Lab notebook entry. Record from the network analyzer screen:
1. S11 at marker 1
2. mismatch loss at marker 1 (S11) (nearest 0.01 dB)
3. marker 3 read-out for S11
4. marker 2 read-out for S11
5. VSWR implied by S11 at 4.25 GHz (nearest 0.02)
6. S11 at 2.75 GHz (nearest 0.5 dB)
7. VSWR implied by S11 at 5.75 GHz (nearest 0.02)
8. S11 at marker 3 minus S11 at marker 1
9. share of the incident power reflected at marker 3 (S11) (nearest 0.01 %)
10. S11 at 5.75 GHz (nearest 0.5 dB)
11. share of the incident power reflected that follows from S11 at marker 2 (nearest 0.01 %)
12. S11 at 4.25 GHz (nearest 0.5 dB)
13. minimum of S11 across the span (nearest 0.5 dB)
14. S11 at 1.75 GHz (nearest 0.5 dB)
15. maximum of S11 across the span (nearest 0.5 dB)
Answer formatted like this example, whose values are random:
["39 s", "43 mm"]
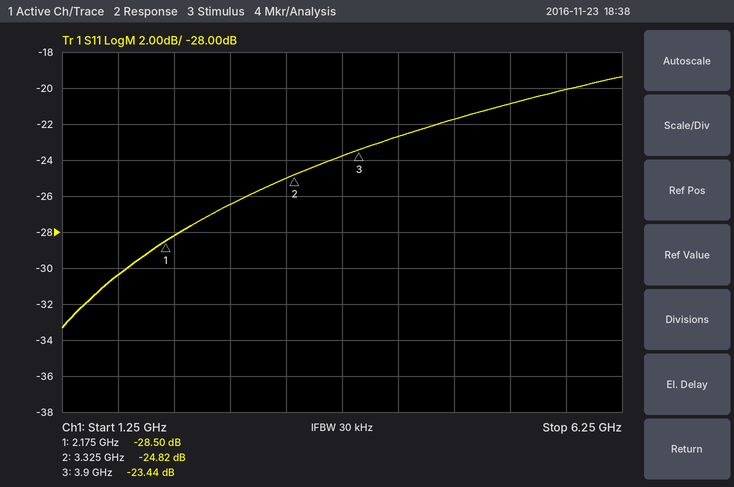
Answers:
["-28.50 dB", "0.01 dB", "-23.44 dB", "-24.82 dB", "1.16", "-26.5 dB", "1.22", "5.06 dB", "0.45 %", "-20.0 dB", "0.33 %", "-22.5 dB", "-33.5 dB", "-30.5 dB", "-19.5 dB"]
